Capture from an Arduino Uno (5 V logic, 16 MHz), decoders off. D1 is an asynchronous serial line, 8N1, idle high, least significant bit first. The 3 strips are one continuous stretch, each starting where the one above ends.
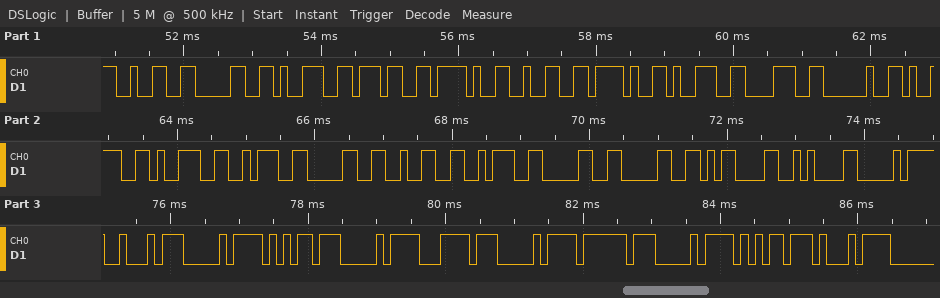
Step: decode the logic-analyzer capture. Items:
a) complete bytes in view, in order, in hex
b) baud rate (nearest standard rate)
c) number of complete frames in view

0x32 0x30 0x39 0x37 0x2F 0x32 0x2F 0x39 0x38 0x20 0x39 0x39 0x3A 0x30 0x32 0x3A 0x30 0x30 0x0D 0x0A 0xD0 0xA2 0xD0 0xB5 0xD0 0xBC 0xD0 0xBF 0xD0 0xB5 0xD1
9600 baud
31
